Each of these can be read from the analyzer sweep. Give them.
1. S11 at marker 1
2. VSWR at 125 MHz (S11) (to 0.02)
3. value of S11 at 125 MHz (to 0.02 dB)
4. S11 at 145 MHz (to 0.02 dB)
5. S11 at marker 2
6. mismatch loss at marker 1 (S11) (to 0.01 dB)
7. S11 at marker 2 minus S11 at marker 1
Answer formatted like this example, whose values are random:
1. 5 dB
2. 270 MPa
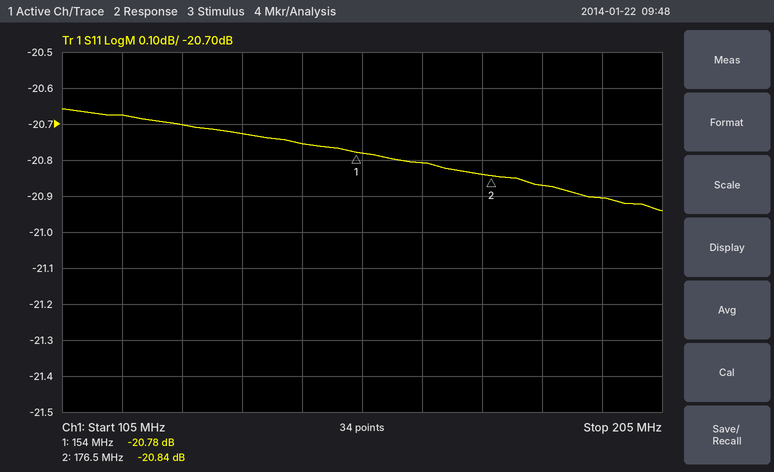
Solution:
1. -20.78 dB
2. 1.20
3. -20.70 dB
4. -20.76 dB
5. -20.84 dB
6. 0.04 dB
7. -0.06 dB
